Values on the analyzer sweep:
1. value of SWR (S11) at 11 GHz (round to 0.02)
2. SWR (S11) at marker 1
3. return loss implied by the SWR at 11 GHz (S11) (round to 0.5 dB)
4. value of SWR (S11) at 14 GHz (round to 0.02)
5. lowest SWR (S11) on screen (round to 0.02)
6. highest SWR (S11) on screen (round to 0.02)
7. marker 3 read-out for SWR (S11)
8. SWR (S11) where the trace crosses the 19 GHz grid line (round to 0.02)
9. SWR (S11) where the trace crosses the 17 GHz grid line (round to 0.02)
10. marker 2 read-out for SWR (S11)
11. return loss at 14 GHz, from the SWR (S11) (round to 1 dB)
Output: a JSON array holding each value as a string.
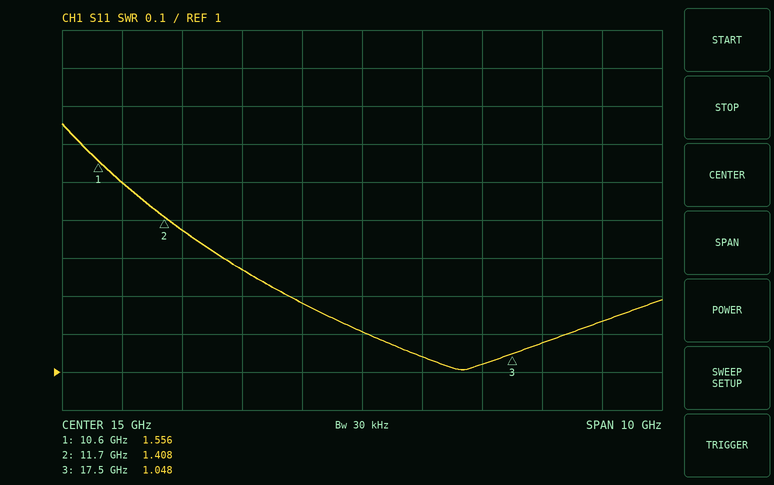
["1.50", "1.556", "14.0 dB", "1.18", "1.00", "1.66", "1.048", "1.14", "1.02", "1.408", "22 dB"]
